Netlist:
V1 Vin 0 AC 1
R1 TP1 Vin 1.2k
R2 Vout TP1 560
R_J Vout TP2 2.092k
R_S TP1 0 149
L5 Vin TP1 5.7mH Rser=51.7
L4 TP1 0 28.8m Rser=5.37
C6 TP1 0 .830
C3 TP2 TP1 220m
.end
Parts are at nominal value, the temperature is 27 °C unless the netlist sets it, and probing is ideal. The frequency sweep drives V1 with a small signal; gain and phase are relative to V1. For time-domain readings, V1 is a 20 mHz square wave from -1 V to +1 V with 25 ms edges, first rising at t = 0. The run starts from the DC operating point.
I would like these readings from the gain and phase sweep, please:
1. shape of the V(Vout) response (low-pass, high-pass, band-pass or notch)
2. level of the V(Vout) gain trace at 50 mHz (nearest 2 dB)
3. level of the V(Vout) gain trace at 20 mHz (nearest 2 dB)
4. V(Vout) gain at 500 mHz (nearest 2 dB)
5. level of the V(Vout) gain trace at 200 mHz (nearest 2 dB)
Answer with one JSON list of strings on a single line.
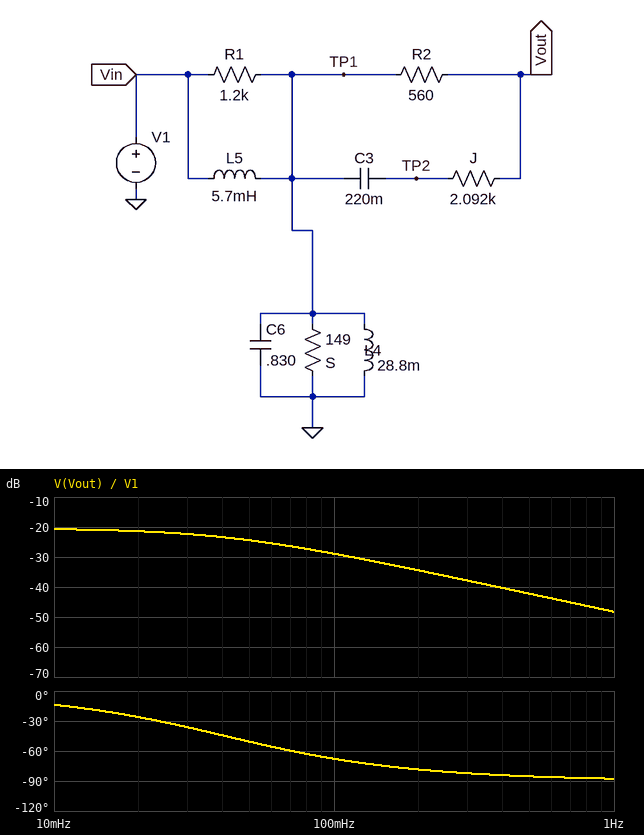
["low-pass", "-24 dB", "-22 dB", "-42 dB", "-34 dB"]
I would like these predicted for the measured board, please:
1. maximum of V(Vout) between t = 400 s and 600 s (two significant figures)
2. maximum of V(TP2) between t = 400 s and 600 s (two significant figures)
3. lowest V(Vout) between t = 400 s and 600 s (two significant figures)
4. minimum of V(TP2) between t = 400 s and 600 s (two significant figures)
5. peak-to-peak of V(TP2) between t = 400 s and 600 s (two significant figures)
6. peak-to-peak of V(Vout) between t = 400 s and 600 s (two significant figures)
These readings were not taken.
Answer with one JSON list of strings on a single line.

["94 mV", "94 mV", "-94 mV", "-94 mV", "190 mV", "190 mV"]
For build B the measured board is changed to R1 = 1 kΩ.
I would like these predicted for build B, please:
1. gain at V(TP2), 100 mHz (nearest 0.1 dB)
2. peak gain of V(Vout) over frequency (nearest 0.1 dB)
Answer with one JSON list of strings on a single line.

["-28.8 dB", "-20.4 dB"]
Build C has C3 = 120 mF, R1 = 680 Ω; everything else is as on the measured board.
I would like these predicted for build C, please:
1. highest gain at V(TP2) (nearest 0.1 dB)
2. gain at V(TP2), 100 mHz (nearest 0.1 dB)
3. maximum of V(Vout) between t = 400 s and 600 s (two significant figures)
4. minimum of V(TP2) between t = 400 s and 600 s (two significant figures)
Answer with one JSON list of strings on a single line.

["-20.2 dB", "-28.6 dB", "97 mV", "-97 mV"]
